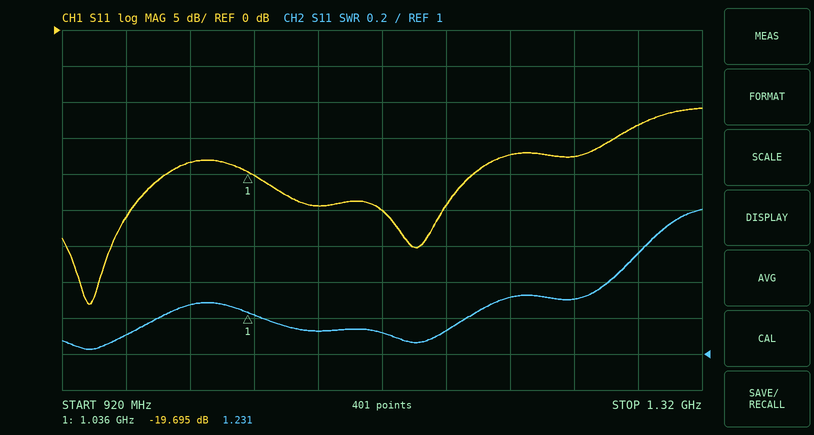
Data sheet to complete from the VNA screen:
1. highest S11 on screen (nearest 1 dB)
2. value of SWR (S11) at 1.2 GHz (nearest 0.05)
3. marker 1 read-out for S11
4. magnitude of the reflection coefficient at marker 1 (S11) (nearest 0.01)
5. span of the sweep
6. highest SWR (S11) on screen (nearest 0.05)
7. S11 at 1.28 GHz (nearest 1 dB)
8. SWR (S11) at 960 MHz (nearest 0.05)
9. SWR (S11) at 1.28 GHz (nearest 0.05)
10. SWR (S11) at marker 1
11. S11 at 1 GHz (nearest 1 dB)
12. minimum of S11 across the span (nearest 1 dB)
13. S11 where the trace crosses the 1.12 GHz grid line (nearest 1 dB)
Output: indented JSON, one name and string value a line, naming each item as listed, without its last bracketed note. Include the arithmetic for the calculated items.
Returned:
{
  "highest S11 on screen": "-11 dB",
  "value of SWR (S11) at 1.2 GHz": "1.30",
  "marker 1 read-out for S11": "-19.695 dB",
  "magnitude of the reflection coefficient at marker 1 (S11)": "10^(-19.695/20) ≈ 0.10",
  "span of the sweep": "400 MHz",
  "highest SWR (S11) on screen": "1.80",
  "S11 at 1.28 GHz": "-13 dB",
  "SWR (S11) at 960 MHz": "1.10",
  "SWR (S11) at 1.28 GHz": "1.55",
  "SWR (S11) at marker 1": "1.231",
  "S11 at 1 GHz": "-18 dB",
  "minimum of S11 across the span": "-38 dB",
  "S11 where the trace crosses the 1.12 GHz grid line": "-25 dB"
}
